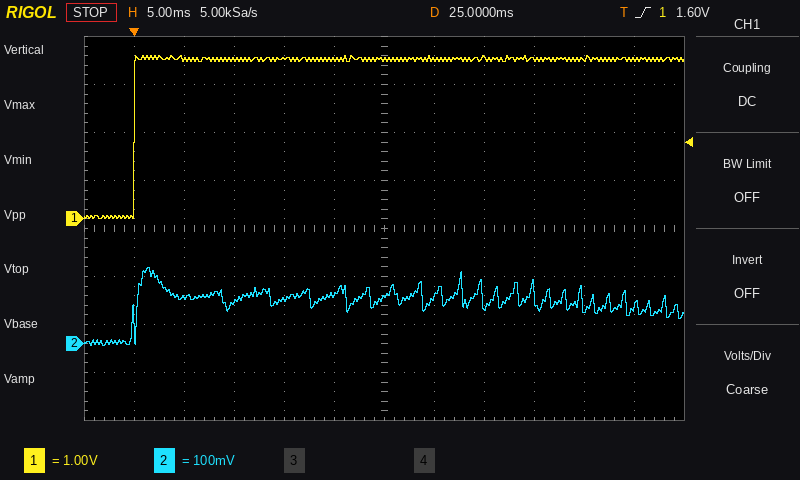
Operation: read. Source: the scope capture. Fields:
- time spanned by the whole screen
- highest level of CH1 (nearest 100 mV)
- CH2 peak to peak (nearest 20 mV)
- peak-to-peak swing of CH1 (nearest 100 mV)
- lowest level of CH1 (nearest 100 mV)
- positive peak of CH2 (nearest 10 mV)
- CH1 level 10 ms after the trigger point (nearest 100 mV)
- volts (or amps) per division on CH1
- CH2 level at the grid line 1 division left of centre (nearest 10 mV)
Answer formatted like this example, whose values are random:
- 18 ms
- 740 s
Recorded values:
- 60 ms
- 3.4 V
- 160 mV
- 3.4 V
- 0.0 V
- 160 mV
- 3.3 V
- 1 V
- 100 mV
